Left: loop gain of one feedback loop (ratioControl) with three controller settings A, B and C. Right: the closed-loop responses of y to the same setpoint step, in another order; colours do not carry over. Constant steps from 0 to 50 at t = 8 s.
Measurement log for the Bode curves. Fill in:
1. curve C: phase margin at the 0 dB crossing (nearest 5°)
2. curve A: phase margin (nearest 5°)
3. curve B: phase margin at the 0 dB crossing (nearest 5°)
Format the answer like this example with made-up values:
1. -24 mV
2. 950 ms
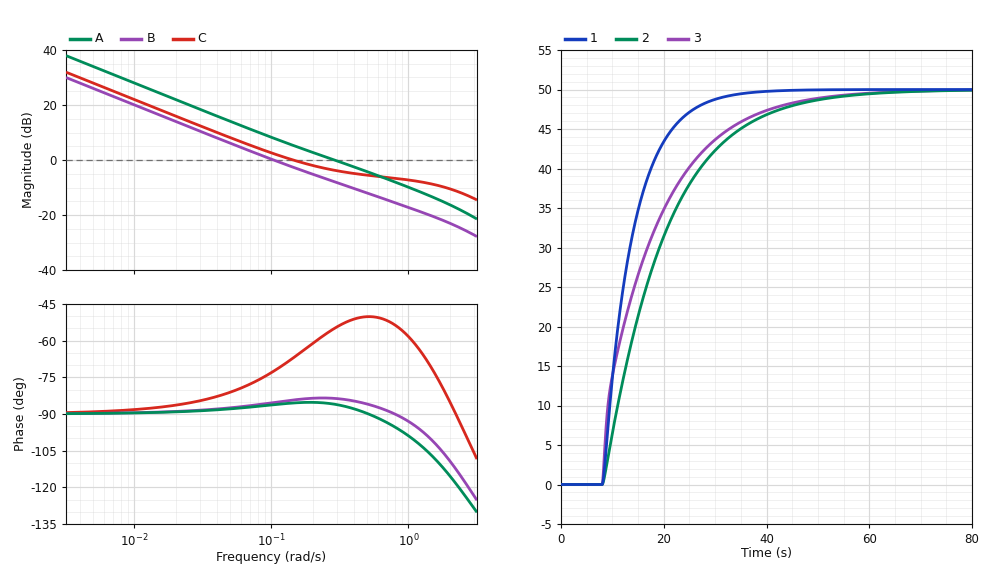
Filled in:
1. 115°
2. 95°
3. 95°
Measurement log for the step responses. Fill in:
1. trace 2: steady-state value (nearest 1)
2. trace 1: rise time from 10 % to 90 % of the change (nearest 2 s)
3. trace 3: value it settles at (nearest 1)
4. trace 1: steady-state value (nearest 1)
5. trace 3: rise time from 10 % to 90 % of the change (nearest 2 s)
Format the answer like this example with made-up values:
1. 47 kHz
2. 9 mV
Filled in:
1. 50
2. 12 s
3. 50
4. 50
5. 24 s
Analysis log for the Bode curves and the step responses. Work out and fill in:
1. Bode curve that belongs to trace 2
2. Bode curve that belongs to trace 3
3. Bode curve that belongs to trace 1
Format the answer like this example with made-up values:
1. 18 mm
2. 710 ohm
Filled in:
1. B
2. C
3. A
